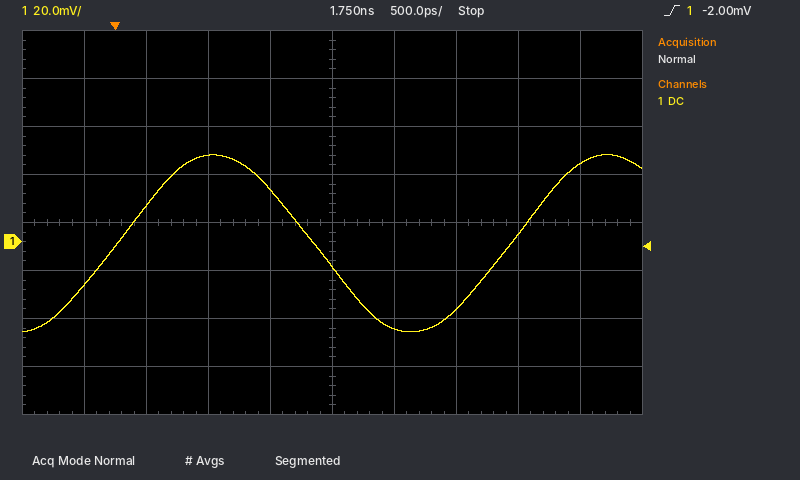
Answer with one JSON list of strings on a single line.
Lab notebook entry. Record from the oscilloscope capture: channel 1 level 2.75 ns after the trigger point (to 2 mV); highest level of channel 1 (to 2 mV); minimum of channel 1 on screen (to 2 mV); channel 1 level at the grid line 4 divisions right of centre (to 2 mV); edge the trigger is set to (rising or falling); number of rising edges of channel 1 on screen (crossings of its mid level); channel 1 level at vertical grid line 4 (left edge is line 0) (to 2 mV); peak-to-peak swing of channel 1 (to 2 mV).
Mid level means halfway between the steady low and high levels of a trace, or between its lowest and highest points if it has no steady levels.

["-28 mV", "36 mV", "-38 mV", "32 mV", "rising", "2", "22 mV", "74 mV"]
